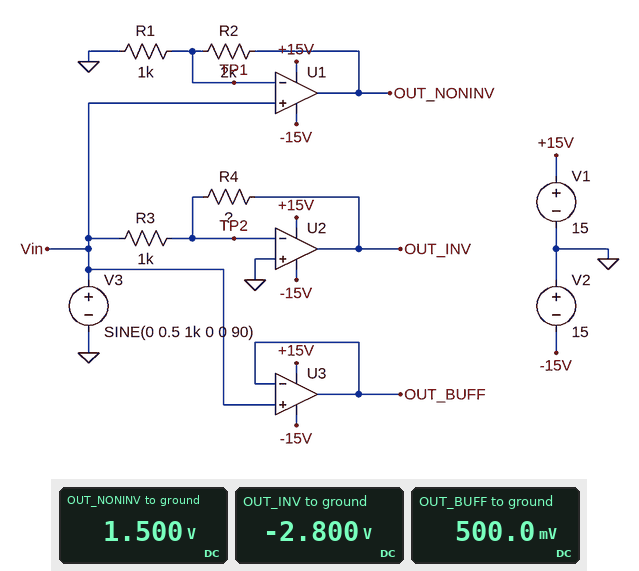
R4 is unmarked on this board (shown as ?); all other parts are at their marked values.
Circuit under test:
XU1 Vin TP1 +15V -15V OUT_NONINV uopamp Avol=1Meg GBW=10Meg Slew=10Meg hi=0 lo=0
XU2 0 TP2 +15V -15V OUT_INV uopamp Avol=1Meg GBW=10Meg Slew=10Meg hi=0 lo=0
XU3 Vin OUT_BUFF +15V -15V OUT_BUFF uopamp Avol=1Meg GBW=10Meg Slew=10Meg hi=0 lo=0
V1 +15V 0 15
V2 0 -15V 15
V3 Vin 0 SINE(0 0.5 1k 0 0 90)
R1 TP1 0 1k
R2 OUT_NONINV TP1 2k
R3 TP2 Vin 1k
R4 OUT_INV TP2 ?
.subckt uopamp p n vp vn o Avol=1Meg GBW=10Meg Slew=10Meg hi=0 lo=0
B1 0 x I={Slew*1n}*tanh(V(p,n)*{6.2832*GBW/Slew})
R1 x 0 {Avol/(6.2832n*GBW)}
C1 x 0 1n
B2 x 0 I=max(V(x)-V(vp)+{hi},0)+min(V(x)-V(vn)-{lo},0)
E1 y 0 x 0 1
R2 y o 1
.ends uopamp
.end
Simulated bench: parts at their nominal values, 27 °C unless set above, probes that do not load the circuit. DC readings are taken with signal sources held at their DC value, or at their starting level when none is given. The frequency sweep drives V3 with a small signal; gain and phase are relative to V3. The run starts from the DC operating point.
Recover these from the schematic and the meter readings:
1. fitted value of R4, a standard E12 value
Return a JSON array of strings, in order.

["5.6 kΩ"]
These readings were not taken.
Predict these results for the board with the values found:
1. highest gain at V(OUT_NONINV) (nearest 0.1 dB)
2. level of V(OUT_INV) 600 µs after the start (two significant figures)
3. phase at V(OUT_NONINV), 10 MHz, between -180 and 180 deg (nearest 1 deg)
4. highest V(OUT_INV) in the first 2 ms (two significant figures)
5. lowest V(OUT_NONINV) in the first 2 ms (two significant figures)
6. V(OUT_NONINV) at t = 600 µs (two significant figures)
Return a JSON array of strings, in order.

["9.5 dB", "2.3 V", "-72 deg", "2.8 V", "-1.5 V", "-1.2 V"]
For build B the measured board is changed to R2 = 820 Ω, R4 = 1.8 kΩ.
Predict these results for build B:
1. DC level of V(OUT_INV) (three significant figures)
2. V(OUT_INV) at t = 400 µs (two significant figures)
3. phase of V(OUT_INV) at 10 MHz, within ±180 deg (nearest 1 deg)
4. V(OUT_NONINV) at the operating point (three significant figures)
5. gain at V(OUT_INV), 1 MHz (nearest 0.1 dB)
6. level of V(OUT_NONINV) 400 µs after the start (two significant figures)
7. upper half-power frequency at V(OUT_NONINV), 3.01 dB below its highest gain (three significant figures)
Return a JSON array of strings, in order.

["-900 mV", "730 mV", "110 deg", "910 mV", "4.8 dB", "-740 mV", "5.49 MHz"]
